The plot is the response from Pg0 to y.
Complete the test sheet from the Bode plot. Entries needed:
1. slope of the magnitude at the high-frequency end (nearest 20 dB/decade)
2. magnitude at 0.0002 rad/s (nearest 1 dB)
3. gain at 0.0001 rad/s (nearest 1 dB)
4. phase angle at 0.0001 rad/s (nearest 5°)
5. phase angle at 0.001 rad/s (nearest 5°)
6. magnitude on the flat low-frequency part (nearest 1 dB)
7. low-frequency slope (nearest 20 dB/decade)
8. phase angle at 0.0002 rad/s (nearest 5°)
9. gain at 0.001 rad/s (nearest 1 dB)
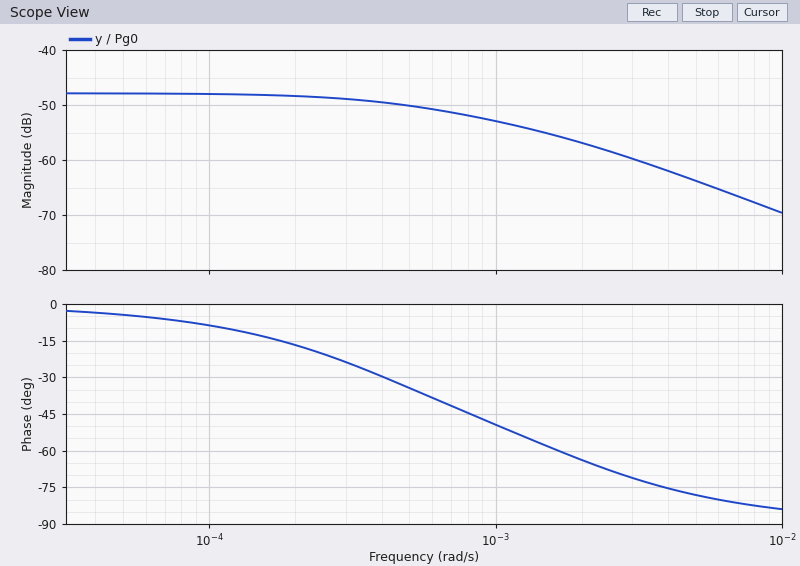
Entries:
-20 dB/decade
-48 dB
-48 dB
-10°
-50°
-48 dB
0 dB/decade
-15°
-53 dB
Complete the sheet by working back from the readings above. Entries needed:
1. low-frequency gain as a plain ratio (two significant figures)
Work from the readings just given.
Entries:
0.0040
